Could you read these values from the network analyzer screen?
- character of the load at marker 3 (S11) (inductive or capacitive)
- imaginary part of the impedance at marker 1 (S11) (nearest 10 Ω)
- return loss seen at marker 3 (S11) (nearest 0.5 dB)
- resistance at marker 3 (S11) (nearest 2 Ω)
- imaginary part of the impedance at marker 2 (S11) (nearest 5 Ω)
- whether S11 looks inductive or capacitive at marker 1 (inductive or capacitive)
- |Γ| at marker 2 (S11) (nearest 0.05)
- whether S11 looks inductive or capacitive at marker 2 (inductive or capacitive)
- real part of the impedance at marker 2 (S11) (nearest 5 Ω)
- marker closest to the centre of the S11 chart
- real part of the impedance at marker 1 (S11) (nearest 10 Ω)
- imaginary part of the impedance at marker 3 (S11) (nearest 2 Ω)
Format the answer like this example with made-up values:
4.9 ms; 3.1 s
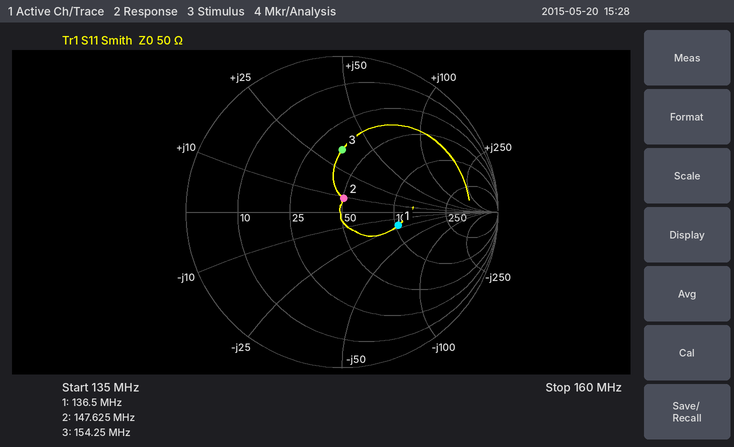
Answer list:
inductive; -20 Ω; 8.0 dB; 36 Ω; +10 Ω; capacitive; 0.10; inductive; 50 Ω; marker 2; 100 Ω; +34 Ω
